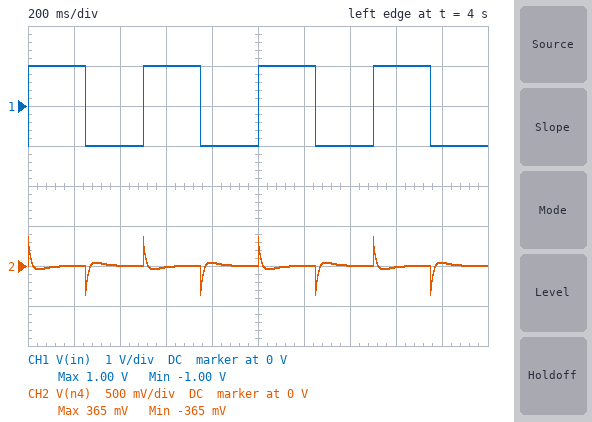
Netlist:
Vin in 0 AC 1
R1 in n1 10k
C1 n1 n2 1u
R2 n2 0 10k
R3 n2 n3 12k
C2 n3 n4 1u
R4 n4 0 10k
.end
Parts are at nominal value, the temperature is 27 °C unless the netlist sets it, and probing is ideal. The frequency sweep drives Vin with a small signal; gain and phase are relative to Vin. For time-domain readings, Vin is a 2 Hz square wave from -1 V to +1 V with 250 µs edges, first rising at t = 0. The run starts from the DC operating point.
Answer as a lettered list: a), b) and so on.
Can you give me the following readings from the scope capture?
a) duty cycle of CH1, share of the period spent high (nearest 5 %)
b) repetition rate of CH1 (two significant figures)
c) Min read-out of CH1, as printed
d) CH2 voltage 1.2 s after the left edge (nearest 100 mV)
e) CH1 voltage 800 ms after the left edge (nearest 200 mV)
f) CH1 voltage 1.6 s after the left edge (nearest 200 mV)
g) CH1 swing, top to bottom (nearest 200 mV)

a) 50 %
b) 2.0 Hz
c) -1.00 V
d) 0 V
e) -1.0 V
f) 1.0 V
g) 2.0 V
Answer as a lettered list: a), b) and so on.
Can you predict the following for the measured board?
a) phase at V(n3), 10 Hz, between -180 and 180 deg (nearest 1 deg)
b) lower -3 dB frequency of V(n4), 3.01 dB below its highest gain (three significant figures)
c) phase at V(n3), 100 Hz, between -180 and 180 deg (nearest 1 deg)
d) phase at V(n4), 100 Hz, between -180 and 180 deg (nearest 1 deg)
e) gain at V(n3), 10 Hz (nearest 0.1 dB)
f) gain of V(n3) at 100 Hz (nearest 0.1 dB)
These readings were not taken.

a) 13 deg
b) 12.5 Hz
c) 0 deg
d) 9 deg
e) -13.4 dB
f) -14.6 dB
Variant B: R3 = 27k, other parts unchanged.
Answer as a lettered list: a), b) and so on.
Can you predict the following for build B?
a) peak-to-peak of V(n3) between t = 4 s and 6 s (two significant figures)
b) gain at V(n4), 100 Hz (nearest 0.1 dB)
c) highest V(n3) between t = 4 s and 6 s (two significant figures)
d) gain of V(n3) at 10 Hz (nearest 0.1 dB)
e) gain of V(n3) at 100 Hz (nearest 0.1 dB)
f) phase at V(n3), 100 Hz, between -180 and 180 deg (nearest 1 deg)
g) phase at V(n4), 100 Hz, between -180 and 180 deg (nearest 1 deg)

a) 510 mV
b) -18.5 dB
c) 260 mV
d) -16.2 dB
e) -18.4 dB
f) -2 deg
g) 7 deg
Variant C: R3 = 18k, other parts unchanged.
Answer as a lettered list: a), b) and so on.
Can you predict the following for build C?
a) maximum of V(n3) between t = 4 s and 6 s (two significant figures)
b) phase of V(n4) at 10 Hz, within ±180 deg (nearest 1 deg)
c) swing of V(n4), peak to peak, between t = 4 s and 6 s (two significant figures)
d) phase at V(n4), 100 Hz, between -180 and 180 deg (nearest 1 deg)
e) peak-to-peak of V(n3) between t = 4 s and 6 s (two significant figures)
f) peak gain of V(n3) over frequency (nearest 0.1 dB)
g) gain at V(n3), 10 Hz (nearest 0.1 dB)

a) 310 mV
b) 66 deg
c) 600 mV
d) 8 deg
e) 620 mV
f) -14.5 dB
g) -14.6 dB
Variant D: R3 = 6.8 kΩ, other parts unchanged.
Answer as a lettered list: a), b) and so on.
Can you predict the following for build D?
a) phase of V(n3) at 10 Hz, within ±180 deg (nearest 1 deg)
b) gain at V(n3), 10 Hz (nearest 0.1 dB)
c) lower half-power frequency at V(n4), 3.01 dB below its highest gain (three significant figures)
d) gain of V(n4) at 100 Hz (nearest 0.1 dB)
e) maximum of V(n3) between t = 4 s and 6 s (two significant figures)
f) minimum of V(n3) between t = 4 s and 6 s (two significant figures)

a) 18 deg
b) -12.2 dB
c) 13.9 Hz
d) -12.9 dB
e) 460 mV
f) -460 mV
